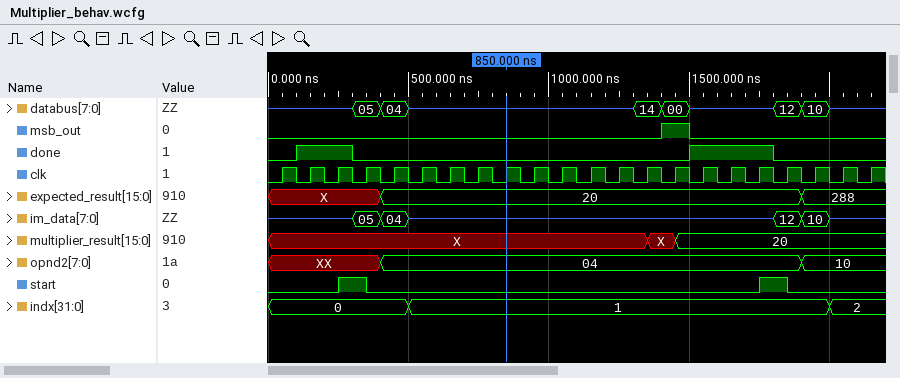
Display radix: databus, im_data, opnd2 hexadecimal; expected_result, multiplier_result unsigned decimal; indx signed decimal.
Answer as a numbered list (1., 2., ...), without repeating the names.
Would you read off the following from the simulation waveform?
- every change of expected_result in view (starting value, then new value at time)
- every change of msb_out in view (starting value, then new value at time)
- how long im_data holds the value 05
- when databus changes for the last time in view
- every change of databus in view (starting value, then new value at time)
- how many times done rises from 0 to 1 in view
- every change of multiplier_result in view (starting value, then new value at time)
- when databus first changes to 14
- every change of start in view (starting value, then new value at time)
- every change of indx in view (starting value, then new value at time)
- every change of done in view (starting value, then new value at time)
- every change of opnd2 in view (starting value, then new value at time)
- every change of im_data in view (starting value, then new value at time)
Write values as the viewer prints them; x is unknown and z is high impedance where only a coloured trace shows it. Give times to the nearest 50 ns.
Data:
1. X, 20 at 400 ns, 288 at 1900 ns
2. 0, 1 at 1400 ns, 0 at 1500 ns
3. 100 ns
4. 2000 ns
5. z, 05 at 300 ns, 04 at 400 ns, z at 500 ns, 14 at 1300 ns, 00 at 1400 ns, z at 1500 ns, 12 at 1800 ns, 10 at 1900 ns, z at 2000 ns
6. 2
7. X, X at 1350 ns, 20 at 1450 ns
8. 1300 ns
9. 0, 1 at 250 ns, 0 at 350 ns, 1 at 1750 ns, 0 at 1850 ns
10. 0, 1 at 500 ns, 2 at 2000 ns
11. 0, 1 at 100 ns, 0 at 300 ns, 1 at 1500 ns, 0 at 1800 ns
12. XX, 04 at 400 ns, 10 at 1900 ns
13. z, 05 at 300 ns, 04 at 400 ns, z at 500 ns, 12 at 1800 ns, 10 at 1900 ns, z at 2000 ns
